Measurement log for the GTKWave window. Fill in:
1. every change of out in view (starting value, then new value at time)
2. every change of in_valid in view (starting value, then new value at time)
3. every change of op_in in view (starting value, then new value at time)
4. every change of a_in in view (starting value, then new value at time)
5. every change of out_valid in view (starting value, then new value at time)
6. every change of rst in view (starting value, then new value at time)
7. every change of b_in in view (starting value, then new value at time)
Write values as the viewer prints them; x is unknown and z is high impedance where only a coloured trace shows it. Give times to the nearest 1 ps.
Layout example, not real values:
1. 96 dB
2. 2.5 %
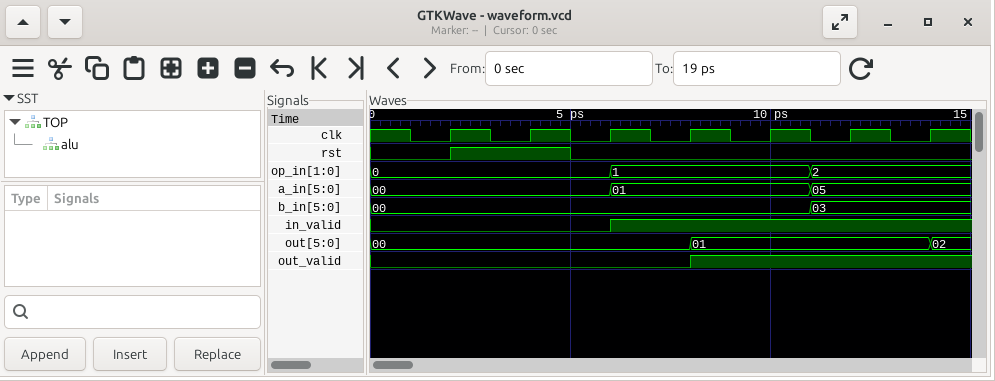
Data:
1. 00, 01 at 8 ps, 02 at 14 ps
2. 0, 1 at 6 ps
3. 0, 1 at 6 ps, 2 at 11 ps
4. 00, 01 at 6 ps, 05 at 11 ps
5. 0, 1 at 8 ps
6. 0, 1 at 2 ps, 0 at 5 ps
7. 00, 03 at 11 ps
